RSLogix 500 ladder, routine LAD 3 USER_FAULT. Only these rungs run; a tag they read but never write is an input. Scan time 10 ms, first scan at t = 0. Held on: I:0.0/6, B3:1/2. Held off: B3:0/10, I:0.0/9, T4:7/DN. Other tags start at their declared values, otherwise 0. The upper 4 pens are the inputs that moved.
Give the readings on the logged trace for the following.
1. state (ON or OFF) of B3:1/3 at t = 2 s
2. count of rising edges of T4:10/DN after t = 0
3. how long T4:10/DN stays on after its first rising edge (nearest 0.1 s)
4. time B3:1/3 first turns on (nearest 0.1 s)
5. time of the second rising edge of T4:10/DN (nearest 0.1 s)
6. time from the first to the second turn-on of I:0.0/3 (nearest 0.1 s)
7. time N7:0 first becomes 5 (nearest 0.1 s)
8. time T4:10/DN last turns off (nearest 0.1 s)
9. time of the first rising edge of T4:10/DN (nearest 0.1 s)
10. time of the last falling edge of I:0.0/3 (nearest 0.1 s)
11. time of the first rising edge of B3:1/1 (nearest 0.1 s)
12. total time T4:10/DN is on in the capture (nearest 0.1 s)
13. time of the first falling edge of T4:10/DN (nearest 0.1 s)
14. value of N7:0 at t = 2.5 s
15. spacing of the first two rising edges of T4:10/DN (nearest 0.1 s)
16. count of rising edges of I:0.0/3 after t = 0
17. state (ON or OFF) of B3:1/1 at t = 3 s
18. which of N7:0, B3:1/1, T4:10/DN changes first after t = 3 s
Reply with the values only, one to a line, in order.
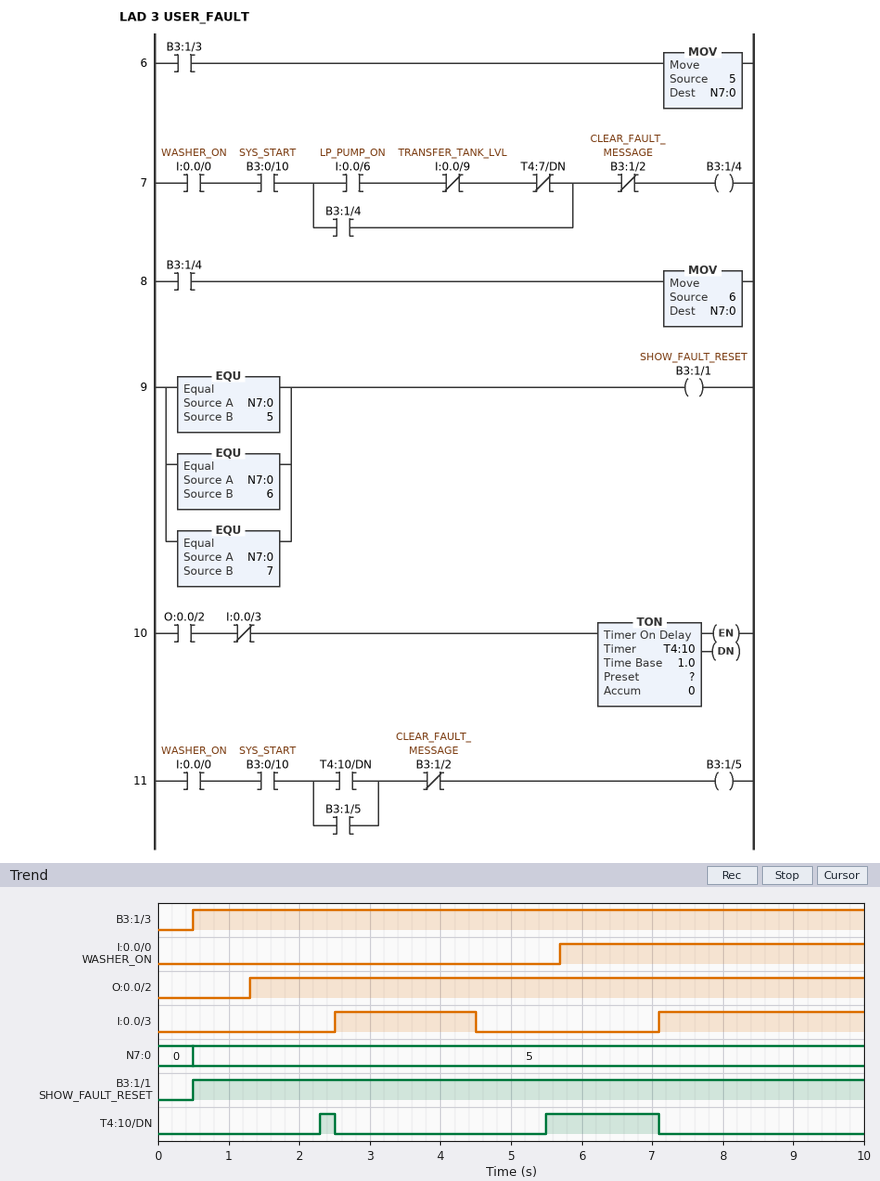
ON
2
0.2 s
0.5 s
5.5 s
4.6 s
0.5 s
7.1 s
2.3 s
4.5 s
0.5 s
1.8 s
2.5 s
5
3.2 s
2
ON
T4:10/DN
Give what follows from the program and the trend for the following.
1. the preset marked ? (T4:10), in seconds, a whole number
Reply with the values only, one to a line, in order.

1 s
